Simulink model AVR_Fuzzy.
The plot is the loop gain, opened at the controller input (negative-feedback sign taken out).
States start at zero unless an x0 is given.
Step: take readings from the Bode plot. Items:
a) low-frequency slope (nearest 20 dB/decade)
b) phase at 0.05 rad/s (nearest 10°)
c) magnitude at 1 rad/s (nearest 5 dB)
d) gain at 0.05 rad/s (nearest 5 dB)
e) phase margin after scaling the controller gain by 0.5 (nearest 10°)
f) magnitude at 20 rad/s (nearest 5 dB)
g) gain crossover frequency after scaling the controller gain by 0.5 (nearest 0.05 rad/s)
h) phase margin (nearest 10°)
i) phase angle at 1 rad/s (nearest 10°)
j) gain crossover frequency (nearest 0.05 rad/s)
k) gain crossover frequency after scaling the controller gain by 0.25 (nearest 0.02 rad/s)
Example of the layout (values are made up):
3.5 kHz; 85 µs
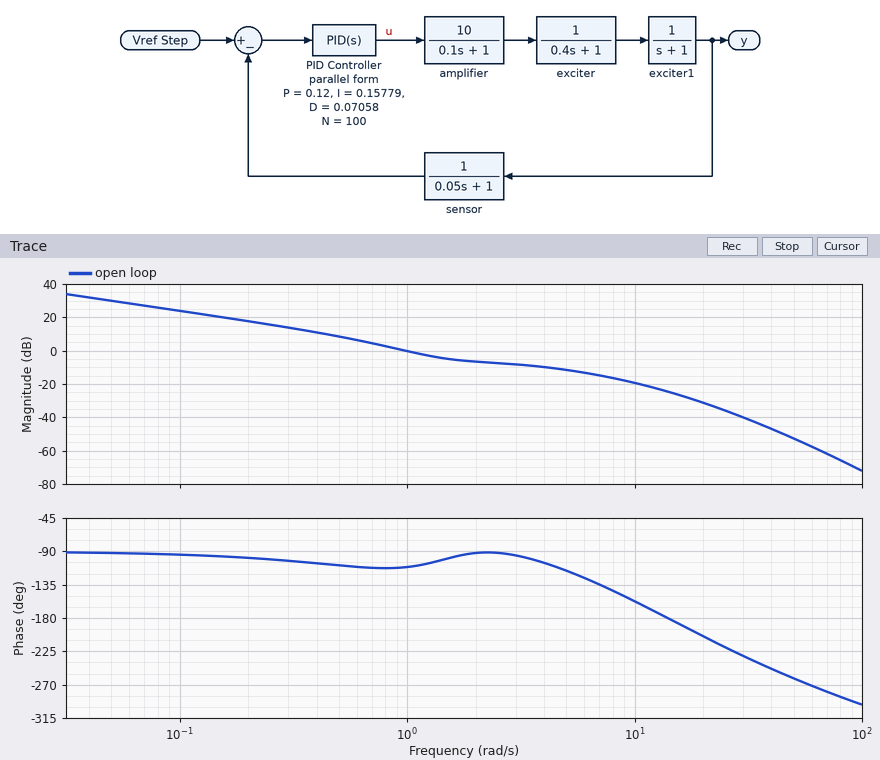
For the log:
-20 dB/decade; -90°; 0 dB; 30 dB; 70°; -30 dB; 0.60 rad/s; 70°; -110°; 1.00 rad/s; 0.36 rad/s
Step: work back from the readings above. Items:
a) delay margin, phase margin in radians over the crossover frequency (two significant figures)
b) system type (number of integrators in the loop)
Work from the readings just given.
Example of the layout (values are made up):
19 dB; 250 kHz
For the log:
1.2 s; 1
